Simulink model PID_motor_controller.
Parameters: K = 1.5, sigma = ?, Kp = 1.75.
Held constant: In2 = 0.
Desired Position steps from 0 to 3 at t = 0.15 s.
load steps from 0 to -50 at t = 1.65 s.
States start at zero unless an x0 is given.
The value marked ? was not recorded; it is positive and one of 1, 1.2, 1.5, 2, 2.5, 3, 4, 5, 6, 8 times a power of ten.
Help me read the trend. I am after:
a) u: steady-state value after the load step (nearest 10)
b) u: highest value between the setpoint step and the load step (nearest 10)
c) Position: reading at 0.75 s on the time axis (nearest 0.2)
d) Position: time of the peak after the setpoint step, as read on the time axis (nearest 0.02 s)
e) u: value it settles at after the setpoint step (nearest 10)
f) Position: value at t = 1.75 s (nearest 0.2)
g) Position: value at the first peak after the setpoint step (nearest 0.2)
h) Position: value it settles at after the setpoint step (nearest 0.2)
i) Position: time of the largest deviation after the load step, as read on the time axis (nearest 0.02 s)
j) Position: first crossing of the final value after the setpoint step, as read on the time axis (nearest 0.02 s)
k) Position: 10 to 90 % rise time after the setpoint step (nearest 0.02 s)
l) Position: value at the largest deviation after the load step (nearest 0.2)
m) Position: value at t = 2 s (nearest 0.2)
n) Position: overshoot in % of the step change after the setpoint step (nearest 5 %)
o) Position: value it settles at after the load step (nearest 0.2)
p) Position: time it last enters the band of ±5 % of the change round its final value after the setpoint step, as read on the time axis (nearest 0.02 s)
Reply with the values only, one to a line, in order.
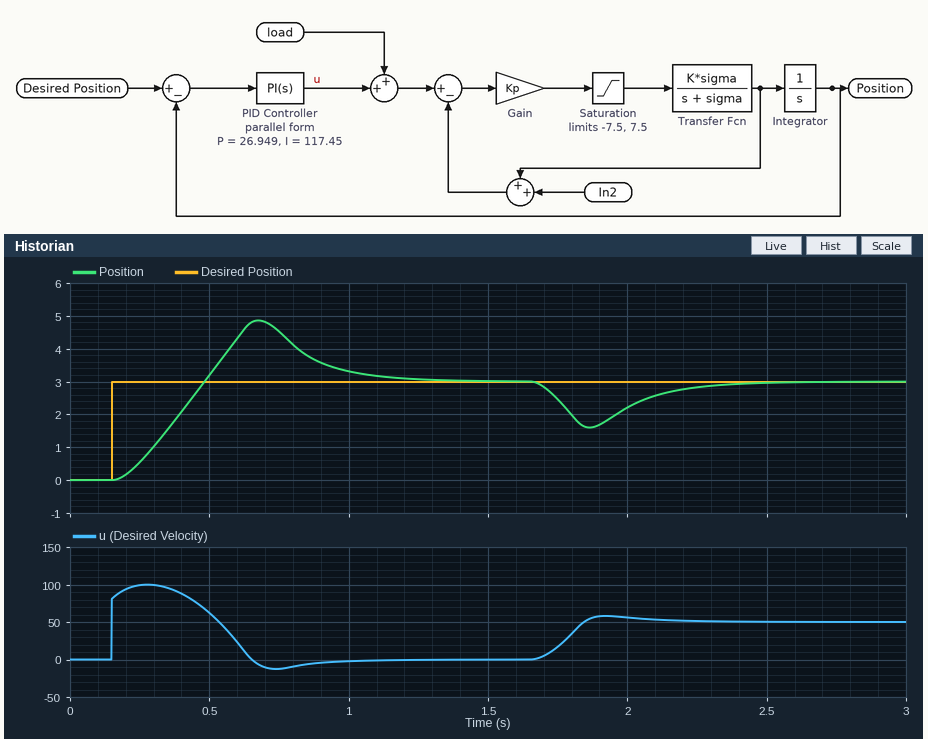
50
100
4.6
0.68 s
0
2.4
4.8
3.0
1.86 s
0.48 s
0.24 s
1.6
2.2
60 %
3.0
1.12 s
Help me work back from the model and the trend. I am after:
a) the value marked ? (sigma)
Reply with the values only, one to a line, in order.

15
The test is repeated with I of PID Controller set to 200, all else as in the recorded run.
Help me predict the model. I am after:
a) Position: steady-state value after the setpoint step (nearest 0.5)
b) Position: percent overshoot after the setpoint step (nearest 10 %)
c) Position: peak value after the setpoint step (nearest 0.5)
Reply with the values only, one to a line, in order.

3.0
80 %
5.5
